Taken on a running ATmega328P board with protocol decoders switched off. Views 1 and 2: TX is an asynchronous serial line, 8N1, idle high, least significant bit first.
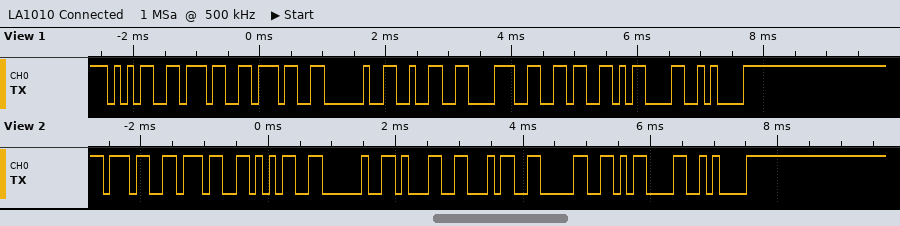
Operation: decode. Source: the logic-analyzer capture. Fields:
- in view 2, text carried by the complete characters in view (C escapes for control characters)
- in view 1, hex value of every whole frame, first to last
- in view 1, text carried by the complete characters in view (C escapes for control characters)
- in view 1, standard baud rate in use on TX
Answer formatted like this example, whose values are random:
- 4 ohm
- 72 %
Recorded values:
- "775 140\r\n"
- 0x35 0x37 0x37 0x20 0x32 0x38 0x36 0x0D 0x0A
- "577 286\r\n"
- 9600 baud
